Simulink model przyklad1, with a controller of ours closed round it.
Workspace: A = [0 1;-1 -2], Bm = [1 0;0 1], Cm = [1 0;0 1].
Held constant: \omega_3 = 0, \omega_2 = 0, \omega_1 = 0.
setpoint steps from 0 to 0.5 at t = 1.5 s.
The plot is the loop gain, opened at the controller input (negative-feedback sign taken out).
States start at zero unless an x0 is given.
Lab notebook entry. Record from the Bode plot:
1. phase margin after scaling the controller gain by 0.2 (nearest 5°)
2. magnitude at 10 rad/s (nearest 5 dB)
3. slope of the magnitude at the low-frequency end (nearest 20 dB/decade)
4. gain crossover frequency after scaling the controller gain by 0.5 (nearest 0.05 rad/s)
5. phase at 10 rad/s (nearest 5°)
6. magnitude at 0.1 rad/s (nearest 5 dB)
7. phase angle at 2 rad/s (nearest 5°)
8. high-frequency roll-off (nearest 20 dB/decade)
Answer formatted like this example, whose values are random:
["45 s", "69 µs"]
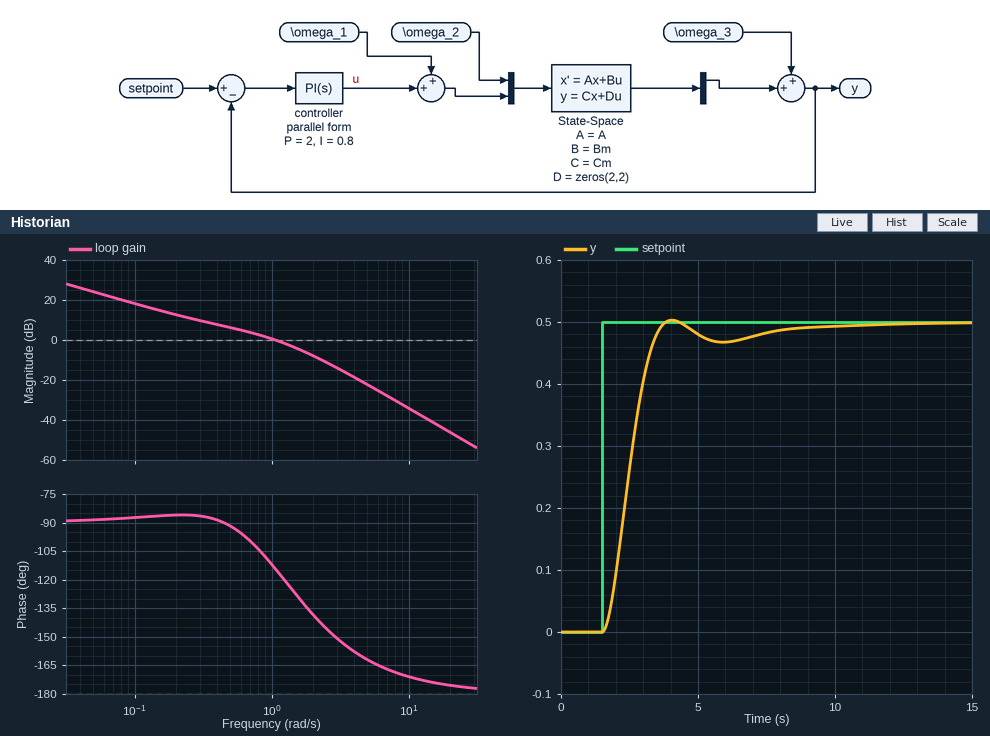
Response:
["95°", "-35 dB", "-20 dB/decade", "0.50 rad/s", "-170°", "20 dB", "-140°", "-40 dB/decade"]
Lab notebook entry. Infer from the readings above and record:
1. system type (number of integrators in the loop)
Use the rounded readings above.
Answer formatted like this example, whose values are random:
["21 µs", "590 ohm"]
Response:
["1"]
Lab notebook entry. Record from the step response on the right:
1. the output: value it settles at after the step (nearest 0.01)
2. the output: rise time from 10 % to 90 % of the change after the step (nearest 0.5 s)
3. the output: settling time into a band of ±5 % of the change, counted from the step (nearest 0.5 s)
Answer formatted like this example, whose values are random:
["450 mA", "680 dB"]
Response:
["0.50", "1.5 s", "5.5 s"]
